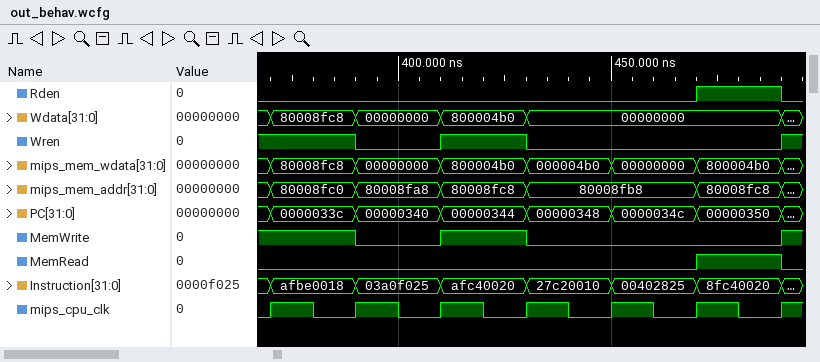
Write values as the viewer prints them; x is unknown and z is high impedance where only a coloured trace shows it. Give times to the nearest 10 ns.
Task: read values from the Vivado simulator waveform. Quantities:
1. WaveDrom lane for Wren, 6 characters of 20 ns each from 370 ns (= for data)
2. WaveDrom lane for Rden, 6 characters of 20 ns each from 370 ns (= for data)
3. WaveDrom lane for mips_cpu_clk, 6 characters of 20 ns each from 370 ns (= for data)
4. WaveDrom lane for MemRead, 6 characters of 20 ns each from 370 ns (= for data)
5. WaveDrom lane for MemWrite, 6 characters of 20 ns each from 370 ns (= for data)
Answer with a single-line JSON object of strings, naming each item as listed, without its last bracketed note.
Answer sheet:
{"WaveDrom lane for Wren, 6 characters of 20 ns each from 370 ns": "{name: 'Wren', wave: '1010..'}", "WaveDrom lane for Rden, 6 characters of 20 ns each from 370 ns": "{name: 'Rden', wave: '0....1'}", "WaveDrom lane for mips_cpu_clk, 6 characters of 20 ns each from 370 ns": "{name: 'mips_cpu_clk', wave: 'p.....'}", "WaveDrom lane for MemRead, 6 characters of 20 ns each from 370 ns": "{name: 'MemRead', wave: '0....1'}", "WaveDrom lane for MemWrite, 6 characters of 20 ns each from 370 ns": "{name: 'MemWrite', wave: '1010..'}"}
